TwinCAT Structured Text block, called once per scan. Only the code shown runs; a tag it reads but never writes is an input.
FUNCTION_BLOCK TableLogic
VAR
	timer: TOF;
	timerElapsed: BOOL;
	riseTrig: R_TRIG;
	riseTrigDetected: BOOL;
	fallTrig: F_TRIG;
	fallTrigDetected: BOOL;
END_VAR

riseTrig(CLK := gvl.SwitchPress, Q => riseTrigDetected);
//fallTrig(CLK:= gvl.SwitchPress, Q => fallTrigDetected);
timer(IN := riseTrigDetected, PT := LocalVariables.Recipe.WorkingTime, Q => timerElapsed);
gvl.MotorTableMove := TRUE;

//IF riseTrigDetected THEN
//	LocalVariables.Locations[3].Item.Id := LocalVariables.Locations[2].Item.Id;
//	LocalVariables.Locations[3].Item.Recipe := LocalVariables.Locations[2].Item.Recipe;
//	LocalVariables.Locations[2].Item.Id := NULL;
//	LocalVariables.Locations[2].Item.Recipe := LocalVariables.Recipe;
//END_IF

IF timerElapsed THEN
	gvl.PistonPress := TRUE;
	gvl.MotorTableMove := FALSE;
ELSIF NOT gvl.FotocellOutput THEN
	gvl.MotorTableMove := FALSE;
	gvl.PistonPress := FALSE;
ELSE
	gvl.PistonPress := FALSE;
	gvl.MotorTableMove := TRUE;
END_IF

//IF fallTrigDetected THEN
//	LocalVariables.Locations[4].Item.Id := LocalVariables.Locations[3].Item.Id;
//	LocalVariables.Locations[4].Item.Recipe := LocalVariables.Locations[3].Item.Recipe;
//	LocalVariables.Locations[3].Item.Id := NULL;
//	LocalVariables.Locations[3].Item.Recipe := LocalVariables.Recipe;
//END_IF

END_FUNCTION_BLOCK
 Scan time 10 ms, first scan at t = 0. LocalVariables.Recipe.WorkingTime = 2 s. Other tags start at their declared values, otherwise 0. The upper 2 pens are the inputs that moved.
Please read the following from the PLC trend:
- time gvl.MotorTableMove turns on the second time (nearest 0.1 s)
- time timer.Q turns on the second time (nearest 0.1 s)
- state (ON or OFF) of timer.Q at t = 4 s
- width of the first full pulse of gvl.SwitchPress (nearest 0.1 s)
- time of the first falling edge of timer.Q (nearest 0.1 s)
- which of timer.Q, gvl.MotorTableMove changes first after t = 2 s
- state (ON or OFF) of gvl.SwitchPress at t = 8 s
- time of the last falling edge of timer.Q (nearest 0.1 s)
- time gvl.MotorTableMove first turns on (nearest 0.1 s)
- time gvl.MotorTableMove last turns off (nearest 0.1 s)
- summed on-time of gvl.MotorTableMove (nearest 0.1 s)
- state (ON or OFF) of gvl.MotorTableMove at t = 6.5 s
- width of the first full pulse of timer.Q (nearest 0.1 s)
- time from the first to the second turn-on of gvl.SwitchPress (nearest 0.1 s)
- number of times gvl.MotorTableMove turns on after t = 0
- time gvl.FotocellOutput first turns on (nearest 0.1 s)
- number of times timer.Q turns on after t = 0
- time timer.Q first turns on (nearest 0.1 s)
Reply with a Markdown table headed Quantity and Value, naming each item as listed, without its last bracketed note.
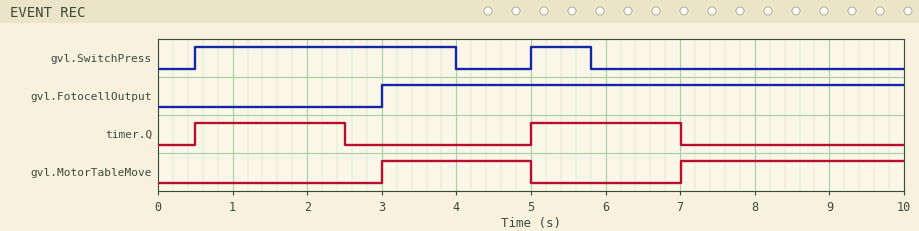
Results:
| Quantity | Value |
|---|---|
| time gvl.MotorTableMove turns on the second time | 7.0 s |
| time timer.Q turns on the second time | 5.0 s |
| state (ON or OFF) of timer.Q at t = 4 s | OFF |
| width of the first full pulse of gvl.SwitchPress | 3.5 s |
| time of the first falling edge of timer.Q | 2.5 s |
| which of timer.Q, gvl.MotorTableMove changes first after t = 2 s | timer.Q |
| state (ON or OFF) of gvl.SwitchPress at t = 8 s | OFF |
| time of the last falling edge of timer.Q | 7.0 s |
| time gvl.MotorTableMove first turns on | 3.0 s |
| time gvl.MotorTableMove last turns off | 5.0 s |
| summed on-time of gvl.MotorTableMove | 5.0 s |
| state (ON or OFF) of gvl.MotorTableMove at t = 6.5 s | OFF |
| width of the first full pulse of timer.Q | 2.0 s |
| time from the first to the second turn-on of gvl.SwitchPress | 4.5 s |
| number of times gvl.MotorTableMove turns on after t = 0 | 2 |
| time gvl.FotocellOutput first turns on | 3.0 s |
| number of times timer.Q turns on after t = 0 | 2 |
| time timer.Q first turns on | 0.5 s |
